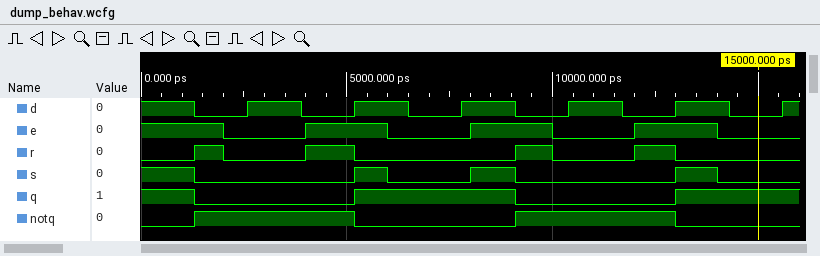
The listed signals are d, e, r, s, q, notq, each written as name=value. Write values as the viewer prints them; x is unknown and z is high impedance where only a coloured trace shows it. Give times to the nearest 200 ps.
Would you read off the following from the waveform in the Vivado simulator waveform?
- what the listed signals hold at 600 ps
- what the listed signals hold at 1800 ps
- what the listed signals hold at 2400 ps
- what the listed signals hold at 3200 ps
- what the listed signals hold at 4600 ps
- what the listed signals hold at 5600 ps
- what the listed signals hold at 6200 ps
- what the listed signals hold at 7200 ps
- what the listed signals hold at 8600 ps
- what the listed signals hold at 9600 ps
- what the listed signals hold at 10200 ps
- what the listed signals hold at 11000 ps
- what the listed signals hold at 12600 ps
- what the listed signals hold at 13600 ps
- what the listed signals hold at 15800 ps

d=1, e=1, r=0, s=1, q=1, notq=0
d=0, e=1, r=1, s=0, q=0, notq=1
d=0, e=0, r=0, s=0, q=0, notq=1
d=1, e=0, r=0, s=0, q=0, notq=1
d=0, e=1, r=1, s=0, q=0, notq=1
d=1, e=1, r=0, s=1, q=1, notq=0
d=1, e=0, r=0, s=0, q=1, notq=0
d=0, e=0, r=0, s=0, q=1, notq=0
d=1, e=1, r=0, s=1, q=1, notq=0
d=0, e=1, r=1, s=0, q=0, notq=1
d=0, e=0, r=0, s=0, q=0, notq=1
d=1, e=0, r=0, s=0, q=0, notq=1
d=0, e=1, r=1, s=0, q=0, notq=1
d=1, e=1, r=0, s=1, q=1, notq=0
d=1, e=0, r=0, s=0, q=1, notq=0
